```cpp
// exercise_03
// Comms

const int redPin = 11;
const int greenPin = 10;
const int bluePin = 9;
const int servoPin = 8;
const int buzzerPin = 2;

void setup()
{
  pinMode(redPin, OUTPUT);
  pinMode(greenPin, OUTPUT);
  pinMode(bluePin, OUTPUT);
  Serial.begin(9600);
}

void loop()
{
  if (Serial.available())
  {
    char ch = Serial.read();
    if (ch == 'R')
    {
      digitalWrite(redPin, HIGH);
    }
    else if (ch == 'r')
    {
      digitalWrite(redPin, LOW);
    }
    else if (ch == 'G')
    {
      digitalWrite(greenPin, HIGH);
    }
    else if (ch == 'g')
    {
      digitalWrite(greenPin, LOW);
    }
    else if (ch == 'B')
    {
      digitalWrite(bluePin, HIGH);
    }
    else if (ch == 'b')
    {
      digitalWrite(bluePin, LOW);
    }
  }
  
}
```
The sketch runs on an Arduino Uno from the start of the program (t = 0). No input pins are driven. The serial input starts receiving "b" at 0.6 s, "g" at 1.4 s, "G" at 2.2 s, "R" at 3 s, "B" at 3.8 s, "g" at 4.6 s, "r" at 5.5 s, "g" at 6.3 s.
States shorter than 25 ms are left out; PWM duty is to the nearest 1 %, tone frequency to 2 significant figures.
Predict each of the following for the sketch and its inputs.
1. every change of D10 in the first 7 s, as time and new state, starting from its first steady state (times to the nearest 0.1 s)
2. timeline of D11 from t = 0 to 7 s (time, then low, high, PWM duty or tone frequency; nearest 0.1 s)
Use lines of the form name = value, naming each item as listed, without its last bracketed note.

every change of D10 in the first 7 s, as time and new state, starting from its first steady state = 0 s low; 2.2 s high; 4.6 s low
timeline of D11 from t = 0 to 7 s = 0 s low; 3 s high; 5.5 s low
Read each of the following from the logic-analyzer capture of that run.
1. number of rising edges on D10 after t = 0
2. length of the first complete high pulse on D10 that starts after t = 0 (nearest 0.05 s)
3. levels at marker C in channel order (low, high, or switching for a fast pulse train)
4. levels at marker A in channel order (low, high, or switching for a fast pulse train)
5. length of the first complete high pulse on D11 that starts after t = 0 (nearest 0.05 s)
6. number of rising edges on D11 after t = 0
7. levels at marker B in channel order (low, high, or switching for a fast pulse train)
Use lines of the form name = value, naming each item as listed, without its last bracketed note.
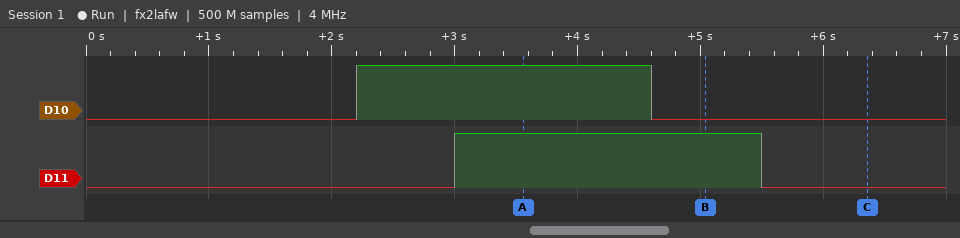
number of rising edges on D10 after t = 0 = 1
length of the first complete high pulse on D10 that starts after t = 0 = 2.40 s
levels at marker C in channel order = D10 low, D11 low
levels at marker A in channel order = D10 high, D11 high
length of the first complete high pulse on D11 that starts after t = 0 = 2.50 s
number of rising edges on D11 after t = 0 = 1
levels at marker B in channel order = D10 low, D11 high
